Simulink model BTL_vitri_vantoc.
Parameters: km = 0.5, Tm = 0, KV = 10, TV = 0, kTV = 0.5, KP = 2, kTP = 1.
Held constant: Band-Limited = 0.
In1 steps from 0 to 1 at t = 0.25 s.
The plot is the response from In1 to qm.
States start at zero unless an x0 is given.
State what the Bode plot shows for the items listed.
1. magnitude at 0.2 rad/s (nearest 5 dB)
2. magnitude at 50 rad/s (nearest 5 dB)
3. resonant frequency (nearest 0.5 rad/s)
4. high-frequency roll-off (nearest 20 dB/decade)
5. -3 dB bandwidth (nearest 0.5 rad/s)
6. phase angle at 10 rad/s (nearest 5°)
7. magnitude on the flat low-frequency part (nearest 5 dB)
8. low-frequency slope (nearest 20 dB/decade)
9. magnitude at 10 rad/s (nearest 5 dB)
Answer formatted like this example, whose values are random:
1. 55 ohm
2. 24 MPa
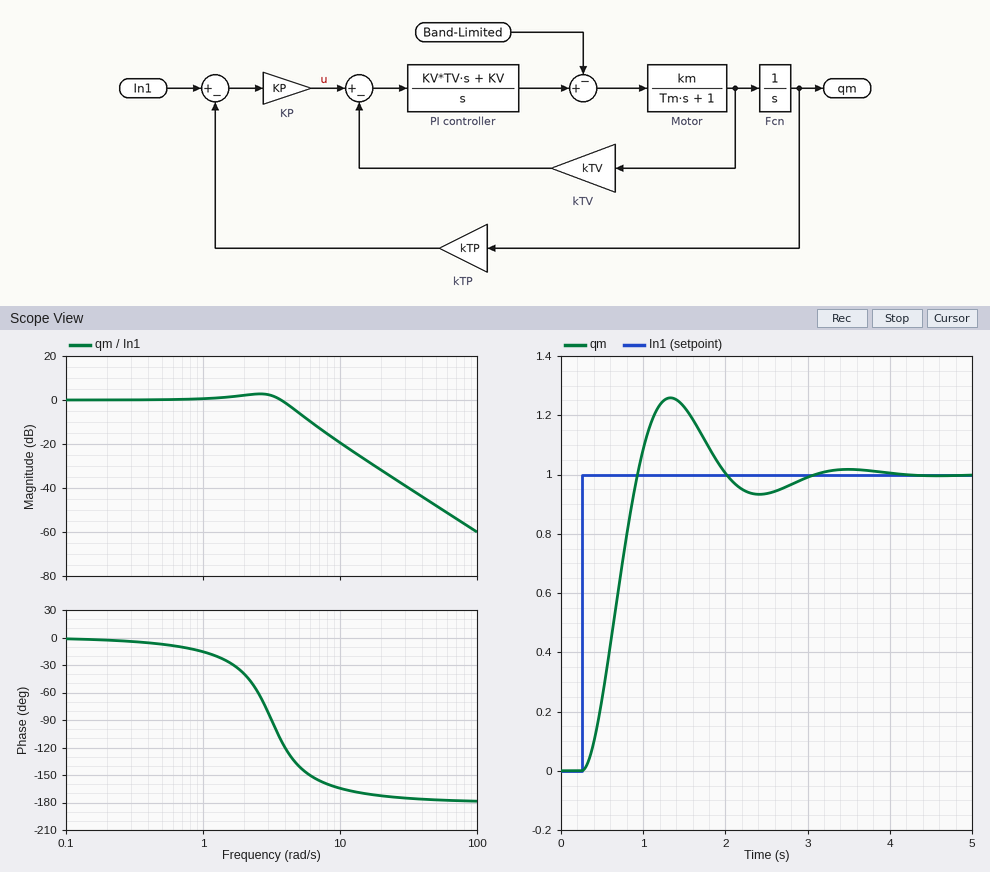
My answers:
1. 0 dB
2. -50 dB
3. 2.5 rad/s
4. -40 dB/decade
5. 4.5 rad/s
6. -165°
7. 0 dB
8. 0 dB/decade
9. -20 dB
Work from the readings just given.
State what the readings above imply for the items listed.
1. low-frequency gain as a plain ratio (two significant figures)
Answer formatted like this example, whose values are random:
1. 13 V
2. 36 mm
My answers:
1. 1.0
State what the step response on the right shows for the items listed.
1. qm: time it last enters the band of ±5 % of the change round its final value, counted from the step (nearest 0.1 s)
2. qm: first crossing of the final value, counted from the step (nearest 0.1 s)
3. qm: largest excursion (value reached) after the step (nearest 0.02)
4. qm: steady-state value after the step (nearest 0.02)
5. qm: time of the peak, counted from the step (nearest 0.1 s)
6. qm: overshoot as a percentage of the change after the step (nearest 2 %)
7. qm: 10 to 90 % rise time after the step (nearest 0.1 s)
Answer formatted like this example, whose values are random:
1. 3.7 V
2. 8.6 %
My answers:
1. 2.4 s
2. 0.7 s
3. 1.26
4. 1.00
5. 1.1 s
6. 26 %
7. 0.5 s
